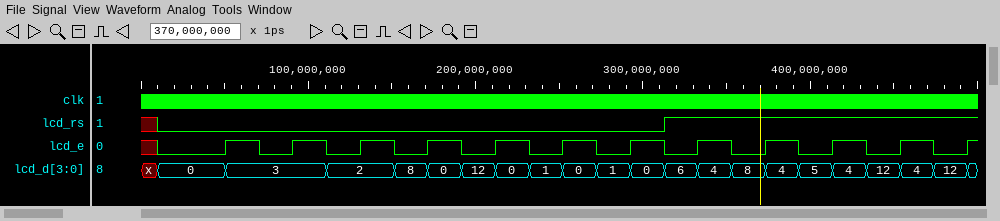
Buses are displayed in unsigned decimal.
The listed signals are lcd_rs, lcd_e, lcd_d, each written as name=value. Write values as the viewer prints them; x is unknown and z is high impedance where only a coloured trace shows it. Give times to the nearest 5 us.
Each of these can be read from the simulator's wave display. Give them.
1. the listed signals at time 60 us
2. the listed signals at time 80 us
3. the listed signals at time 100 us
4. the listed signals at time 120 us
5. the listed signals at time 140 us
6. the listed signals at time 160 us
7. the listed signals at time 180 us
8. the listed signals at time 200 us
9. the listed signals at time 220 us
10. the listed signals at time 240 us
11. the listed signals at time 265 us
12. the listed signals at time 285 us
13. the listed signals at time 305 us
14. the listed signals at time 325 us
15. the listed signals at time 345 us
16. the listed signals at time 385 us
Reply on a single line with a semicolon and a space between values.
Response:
lcd_rs=0, lcd_e=1, lcd_d=3; lcd_rs=0, lcd_e=0, lcd_d=3; lcd_rs=0, lcd_e=1, lcd_d=3; lcd_rs=0, lcd_e=0, lcd_d=2; lcd_rs=0, lcd_e=1, lcd_d=2; lcd_rs=0, lcd_e=0, lcd_d=8; lcd_rs=0, lcd_e=1, lcd_d=0; lcd_rs=0, lcd_e=0, lcd_d=12; lcd_rs=0, lcd_e=1, lcd_d=0; lcd_rs=0, lcd_e=0, lcd_d=1; lcd_rs=0, lcd_e=1, lcd_d=0; lcd_rs=0, lcd_e=0, lcd_d=1; lcd_rs=0, lcd_e=1, lcd_d=0; lcd_rs=1, lcd_e=0, lcd_d=6; lcd_rs=1, lcd_e=1, lcd_d=4; lcd_rs=1, lcd_e=1, lcd_d=4
